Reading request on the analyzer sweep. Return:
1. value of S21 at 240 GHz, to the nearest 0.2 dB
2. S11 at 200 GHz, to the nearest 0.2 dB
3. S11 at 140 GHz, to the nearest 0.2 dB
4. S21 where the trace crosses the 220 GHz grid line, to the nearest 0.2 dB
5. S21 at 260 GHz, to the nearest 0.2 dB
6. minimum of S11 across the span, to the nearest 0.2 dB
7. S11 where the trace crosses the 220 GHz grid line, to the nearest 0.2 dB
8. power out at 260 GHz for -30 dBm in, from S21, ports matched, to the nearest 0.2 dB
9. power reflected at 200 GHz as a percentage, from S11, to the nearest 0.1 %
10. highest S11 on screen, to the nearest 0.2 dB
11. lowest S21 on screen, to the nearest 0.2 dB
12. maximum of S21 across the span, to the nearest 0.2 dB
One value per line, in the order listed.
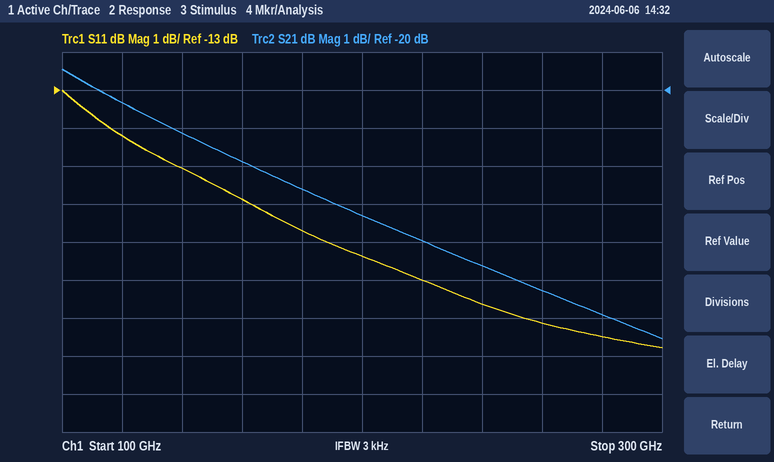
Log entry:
-24.6 dB
-17.4 dB
-15.0 dB
-24.0 dB
-25.2 dB
-19.8 dB
-18.0 dB
-55.2 dBm
1.8 %
-13.0 dB
-26.6 dB
-19.4 dB
